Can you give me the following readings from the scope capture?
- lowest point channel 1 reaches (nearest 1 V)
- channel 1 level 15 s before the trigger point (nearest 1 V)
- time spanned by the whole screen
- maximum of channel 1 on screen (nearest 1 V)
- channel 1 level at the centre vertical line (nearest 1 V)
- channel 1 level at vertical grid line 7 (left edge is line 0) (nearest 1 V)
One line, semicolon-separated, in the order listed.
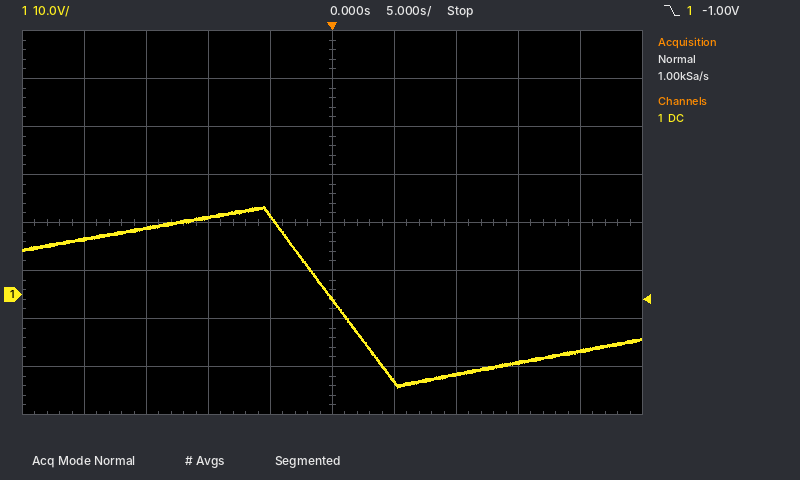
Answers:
-19 V; 14 V; 50 s; 18 V; -1 V; -17 V
